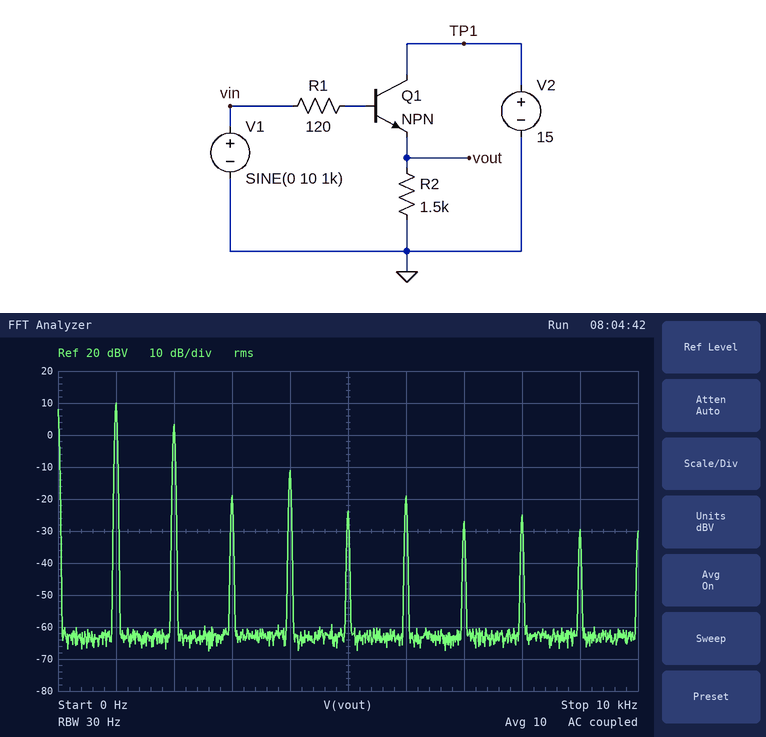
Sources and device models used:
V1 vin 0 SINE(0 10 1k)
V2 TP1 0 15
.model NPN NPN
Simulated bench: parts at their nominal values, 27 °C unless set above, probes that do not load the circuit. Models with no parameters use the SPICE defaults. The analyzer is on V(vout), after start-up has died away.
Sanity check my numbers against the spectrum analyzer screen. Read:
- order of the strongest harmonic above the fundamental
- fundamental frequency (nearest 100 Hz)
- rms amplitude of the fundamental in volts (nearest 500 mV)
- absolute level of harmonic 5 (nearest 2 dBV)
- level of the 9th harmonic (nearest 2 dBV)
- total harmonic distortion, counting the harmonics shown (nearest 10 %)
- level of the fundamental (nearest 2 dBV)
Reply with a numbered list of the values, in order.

1. 2
2. 1.0 kHz
3. 3.0 V
4. -24 dBV
5. -30 dBV
6. 50 %
7. 10 dBV
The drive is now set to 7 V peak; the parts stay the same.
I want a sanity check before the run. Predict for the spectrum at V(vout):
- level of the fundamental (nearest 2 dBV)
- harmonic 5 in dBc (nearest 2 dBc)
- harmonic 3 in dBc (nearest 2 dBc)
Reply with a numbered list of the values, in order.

1. 6 dBV
2. -30 dBc
3. -26 dBc
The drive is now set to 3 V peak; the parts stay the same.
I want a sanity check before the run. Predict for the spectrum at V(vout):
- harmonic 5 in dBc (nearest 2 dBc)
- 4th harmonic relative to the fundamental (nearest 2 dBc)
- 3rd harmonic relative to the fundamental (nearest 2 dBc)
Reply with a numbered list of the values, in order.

1. -24 dBc
2. -24 dBc
3. -18 dBc
